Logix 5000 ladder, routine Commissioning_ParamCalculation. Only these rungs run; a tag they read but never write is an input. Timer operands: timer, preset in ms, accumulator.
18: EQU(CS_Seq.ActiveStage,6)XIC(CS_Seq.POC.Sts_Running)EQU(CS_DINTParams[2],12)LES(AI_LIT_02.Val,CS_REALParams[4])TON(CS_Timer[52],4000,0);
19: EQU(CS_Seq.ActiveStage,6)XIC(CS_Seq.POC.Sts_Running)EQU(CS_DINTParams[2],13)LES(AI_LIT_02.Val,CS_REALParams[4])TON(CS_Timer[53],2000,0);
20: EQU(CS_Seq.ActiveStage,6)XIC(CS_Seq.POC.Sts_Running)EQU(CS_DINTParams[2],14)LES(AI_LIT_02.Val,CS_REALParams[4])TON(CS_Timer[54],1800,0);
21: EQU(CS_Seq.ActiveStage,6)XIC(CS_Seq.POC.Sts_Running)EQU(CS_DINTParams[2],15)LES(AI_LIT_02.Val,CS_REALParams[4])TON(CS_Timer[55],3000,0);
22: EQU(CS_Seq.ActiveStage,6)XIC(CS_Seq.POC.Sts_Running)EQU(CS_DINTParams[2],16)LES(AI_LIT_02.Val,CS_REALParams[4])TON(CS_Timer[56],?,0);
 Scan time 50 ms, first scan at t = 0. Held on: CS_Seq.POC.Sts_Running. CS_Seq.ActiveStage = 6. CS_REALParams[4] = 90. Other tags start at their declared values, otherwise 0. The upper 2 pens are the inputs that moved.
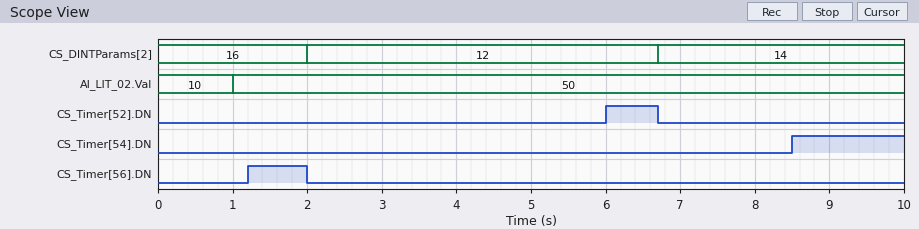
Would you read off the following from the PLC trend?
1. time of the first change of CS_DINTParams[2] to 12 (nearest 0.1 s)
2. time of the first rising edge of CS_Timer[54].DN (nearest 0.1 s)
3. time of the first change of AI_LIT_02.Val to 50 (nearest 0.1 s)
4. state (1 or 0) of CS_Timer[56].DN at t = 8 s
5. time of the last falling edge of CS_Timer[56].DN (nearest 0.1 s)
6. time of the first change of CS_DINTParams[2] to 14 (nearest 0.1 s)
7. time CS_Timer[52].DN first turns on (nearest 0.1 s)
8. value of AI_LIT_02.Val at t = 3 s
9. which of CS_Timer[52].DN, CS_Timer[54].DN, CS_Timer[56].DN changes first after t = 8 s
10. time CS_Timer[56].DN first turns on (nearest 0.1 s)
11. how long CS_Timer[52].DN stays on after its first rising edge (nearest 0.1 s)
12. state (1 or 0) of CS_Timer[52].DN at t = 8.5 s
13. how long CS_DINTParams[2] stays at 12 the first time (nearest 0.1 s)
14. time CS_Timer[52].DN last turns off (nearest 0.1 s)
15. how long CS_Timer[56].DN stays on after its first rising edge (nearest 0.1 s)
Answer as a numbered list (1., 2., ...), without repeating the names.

1. 2.0 s
2. 8.5 s
3. 1.0 s
4. 0
5. 2.0 s
6. 6.7 s
7. 6.0 s
8. 50
9. CS_Timer[54].DN
10. 1.2 s
11. 0.7 s
12. 0
13. 4.7 s
14. 6.7 s
15. 0.8 s
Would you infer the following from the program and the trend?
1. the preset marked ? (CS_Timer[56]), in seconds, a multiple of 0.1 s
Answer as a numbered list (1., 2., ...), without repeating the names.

1. 1.2 s
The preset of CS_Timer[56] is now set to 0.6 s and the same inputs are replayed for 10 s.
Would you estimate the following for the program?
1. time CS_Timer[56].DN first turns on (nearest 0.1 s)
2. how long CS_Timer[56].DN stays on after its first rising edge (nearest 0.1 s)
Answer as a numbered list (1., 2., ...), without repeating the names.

1. 0.6 s
2. 1.4 s
